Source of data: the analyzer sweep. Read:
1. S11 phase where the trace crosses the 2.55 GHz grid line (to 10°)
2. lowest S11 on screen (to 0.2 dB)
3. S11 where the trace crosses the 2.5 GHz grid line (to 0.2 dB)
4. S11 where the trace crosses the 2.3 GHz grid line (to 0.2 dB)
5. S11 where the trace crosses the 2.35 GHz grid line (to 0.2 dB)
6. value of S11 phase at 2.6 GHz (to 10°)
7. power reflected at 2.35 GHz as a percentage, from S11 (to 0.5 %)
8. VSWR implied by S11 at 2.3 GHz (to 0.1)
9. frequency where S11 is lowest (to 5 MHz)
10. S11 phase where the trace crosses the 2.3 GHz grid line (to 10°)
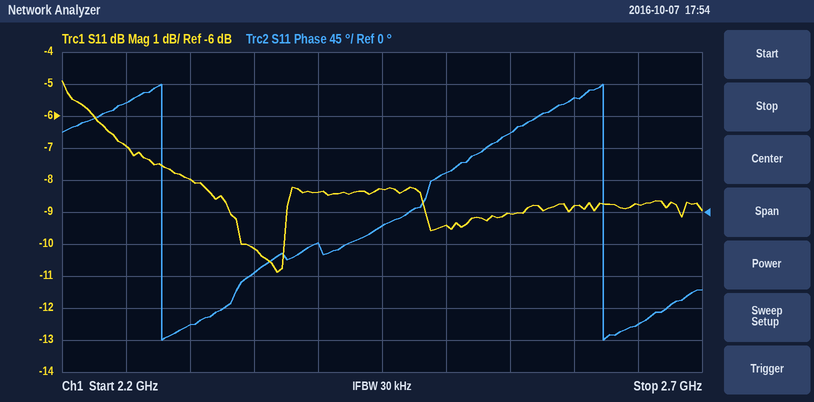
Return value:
110°
-10.8 dB
-9.4 dB
-8.0 dB
-10.2 dB
160°
9.5 %
2.3
2.370 GHz
-160°
